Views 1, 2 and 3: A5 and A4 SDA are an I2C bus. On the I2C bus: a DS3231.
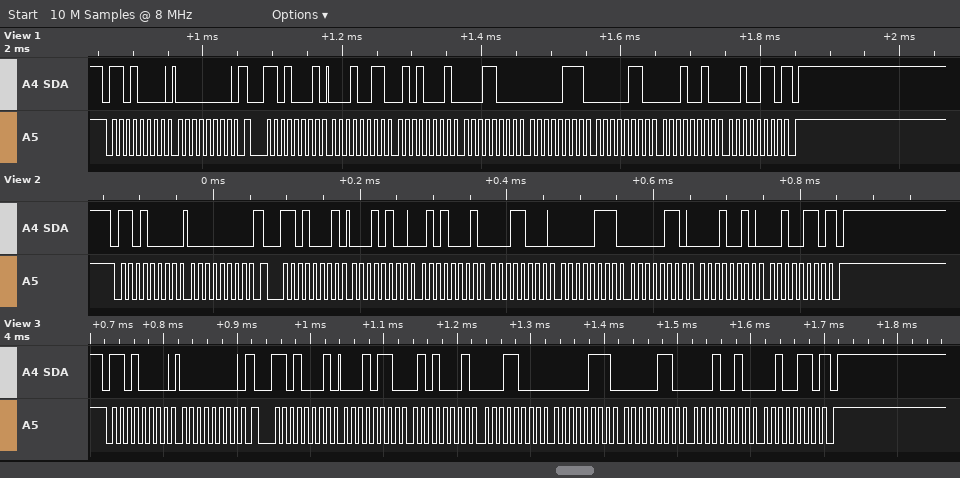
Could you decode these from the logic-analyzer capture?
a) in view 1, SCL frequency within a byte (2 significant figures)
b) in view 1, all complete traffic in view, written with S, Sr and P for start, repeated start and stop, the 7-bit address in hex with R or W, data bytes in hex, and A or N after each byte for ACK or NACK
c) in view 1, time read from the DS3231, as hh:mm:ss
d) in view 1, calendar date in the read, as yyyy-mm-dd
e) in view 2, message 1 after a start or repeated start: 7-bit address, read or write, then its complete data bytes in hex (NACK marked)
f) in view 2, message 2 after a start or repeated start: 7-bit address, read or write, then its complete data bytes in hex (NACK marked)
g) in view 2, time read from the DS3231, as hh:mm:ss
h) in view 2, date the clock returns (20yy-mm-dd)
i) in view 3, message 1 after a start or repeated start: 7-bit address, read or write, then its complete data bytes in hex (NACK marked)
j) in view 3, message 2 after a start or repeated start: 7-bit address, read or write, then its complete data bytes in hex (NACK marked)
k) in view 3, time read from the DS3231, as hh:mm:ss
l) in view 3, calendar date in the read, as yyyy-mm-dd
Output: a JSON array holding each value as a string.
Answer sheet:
["100 kHz", "S 68W A 00 A Sr 68R A 13 A 51 A 18 A 07 A 06 A 12 A 26 N P", "18:51:13", "2026-12-06", "0x68 write: 00", "0x68 read: 14 51 18 07 06 12 26 NACK", "18:51:14", "2026-12-06", "0x68 write: 00", "0x68 read: 16 51 18 07 06 12 26 NACK", "18:51:16", "2026-12-06"]
